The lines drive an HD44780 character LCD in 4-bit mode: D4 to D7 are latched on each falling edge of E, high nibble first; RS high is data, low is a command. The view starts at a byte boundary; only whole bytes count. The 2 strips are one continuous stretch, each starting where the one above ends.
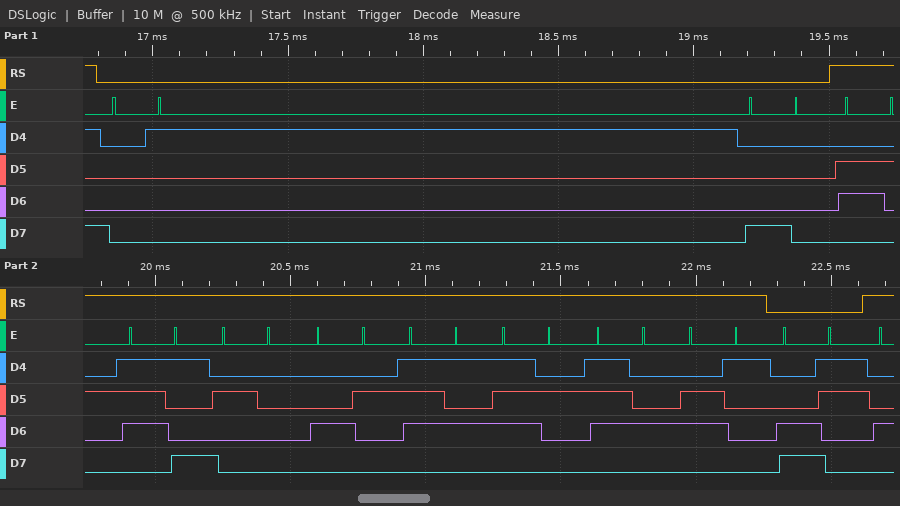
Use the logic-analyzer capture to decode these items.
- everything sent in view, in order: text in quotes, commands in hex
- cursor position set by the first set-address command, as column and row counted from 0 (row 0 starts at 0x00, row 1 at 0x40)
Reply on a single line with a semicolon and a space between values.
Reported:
0x01 0x80 "by Burta" 0xC3; column 0, row 0
